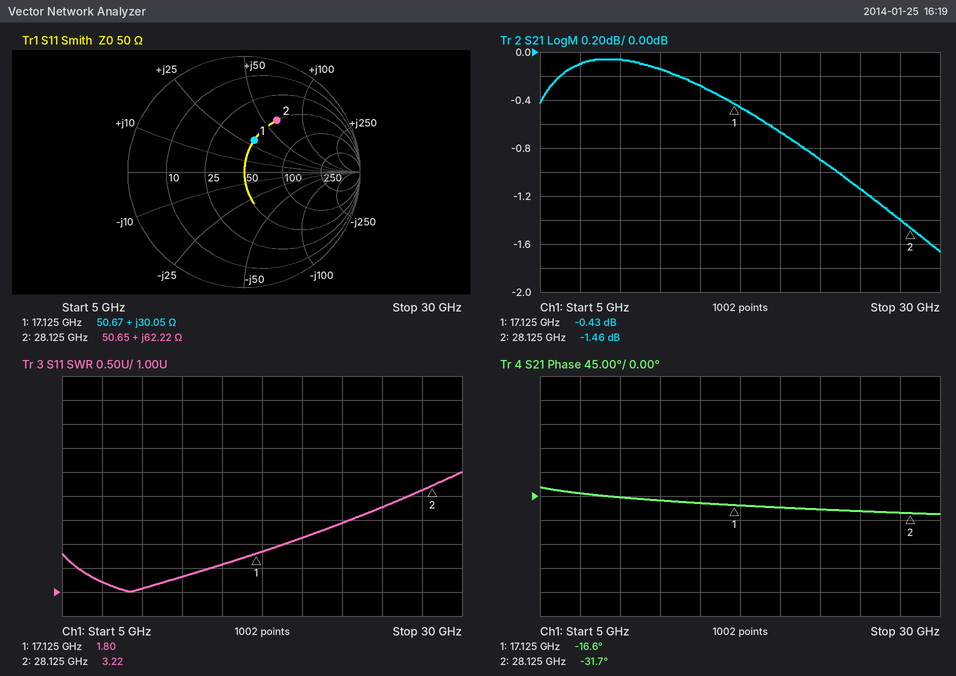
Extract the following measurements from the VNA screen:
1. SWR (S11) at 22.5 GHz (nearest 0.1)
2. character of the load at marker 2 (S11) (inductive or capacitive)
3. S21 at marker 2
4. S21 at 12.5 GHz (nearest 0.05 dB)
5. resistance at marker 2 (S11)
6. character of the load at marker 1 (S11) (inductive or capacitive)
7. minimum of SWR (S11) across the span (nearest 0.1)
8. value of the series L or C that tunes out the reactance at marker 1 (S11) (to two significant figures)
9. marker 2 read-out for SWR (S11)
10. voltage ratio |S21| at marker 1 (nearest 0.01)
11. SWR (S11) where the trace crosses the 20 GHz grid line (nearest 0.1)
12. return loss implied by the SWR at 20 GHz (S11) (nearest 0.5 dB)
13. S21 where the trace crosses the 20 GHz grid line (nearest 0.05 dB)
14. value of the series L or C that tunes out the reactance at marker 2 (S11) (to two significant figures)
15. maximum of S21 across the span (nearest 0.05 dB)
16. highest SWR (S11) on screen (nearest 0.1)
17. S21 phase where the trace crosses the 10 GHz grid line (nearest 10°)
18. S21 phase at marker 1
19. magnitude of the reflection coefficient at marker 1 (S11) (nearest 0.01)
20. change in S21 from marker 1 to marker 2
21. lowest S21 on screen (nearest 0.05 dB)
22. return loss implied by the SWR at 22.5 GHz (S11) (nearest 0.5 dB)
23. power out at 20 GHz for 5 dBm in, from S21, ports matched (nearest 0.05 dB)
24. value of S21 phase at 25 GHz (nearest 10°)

2.4
inductive
-1.46 dB
-0.15 dB
50.65 Ω
inductive
1.0
310 fF
3.22
0.95
2.1
9.0 dB
-0.65 dB
91 fF
-0.05 dB
3.5
0°
-16.6°
0.29
-1.03 dB
-1.65 dB
7.5 dB
4.35 dBm
-30°
